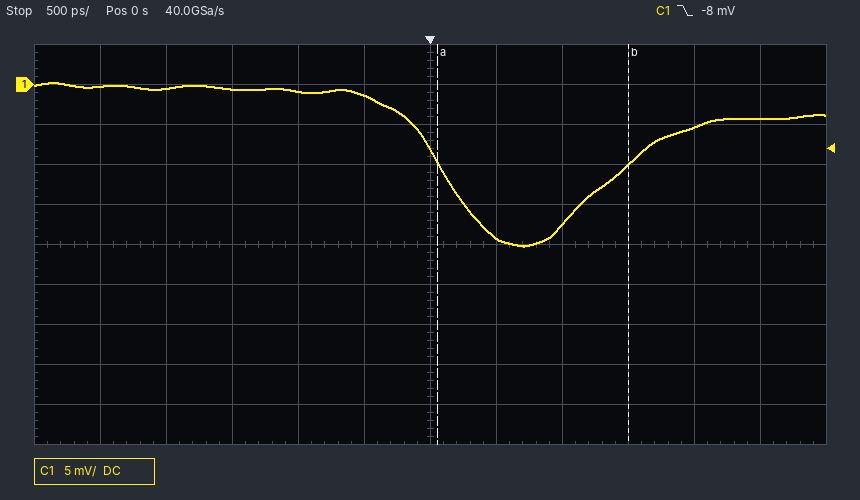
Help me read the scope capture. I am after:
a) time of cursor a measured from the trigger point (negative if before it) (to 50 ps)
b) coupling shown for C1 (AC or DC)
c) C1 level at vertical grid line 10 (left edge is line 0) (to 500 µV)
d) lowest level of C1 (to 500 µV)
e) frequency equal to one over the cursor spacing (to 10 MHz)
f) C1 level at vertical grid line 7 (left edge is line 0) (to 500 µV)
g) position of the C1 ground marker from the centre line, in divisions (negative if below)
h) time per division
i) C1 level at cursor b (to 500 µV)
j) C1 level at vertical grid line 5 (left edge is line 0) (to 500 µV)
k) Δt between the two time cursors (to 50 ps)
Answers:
+50 ps
DC
-5.5 mV
-20.0 mV
690 MHz
-19.0 mV
+4.0 div
500 ps
-10.0 mV
-1.5 mV
1.45 ns
